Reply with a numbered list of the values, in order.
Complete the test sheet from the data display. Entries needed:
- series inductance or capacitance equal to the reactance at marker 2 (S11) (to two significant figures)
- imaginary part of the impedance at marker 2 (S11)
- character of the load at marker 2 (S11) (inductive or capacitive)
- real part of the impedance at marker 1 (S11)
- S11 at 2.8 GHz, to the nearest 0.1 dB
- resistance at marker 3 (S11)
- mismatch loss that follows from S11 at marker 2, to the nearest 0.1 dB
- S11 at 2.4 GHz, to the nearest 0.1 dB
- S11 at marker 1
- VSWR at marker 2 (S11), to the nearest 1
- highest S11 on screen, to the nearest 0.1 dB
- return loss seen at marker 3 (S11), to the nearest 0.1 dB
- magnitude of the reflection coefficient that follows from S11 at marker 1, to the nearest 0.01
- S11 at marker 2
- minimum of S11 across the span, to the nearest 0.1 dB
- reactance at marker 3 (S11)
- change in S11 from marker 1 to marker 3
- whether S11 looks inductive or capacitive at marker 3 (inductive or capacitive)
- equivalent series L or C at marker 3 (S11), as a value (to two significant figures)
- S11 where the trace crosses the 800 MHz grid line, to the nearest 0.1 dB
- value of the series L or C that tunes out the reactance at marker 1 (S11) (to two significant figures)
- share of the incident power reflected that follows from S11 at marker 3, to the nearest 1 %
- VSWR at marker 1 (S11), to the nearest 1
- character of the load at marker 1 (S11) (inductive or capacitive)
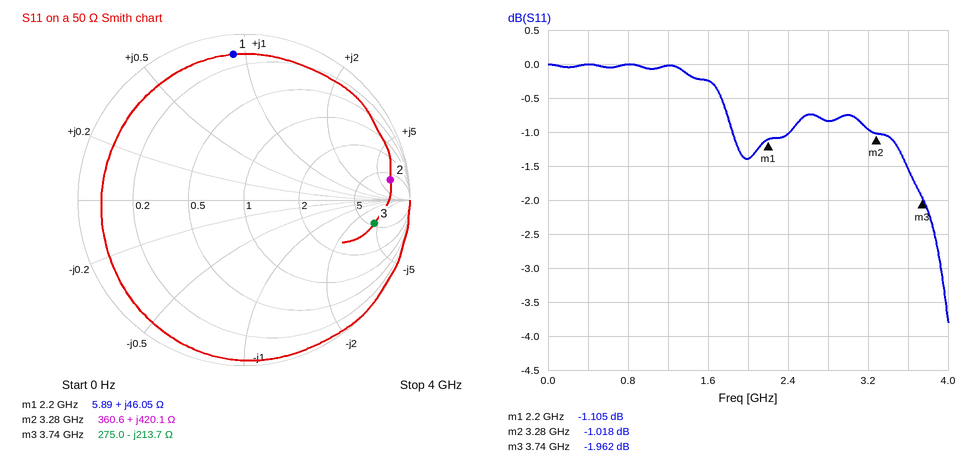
1. 20 nH
2. +420.1 Ω
3. inductive
4. 5.89 Ω
5. -0.8 dB
6. 275.0 Ω
7. 6.8 dB
8. -1.0 dB
9. -1.105 dB
10. 17
11. 0.0 dB
12. 2.0 dB
13. 0.88
14. -1.018 dB
15. -3.8 dB
16. -213.7 Ω
17. -0.857 dB
18. capacitive
19. 200 fF
20. 0.0 dB
21. 1.6 pF
22. 64 %
23. 16
24. inductive
